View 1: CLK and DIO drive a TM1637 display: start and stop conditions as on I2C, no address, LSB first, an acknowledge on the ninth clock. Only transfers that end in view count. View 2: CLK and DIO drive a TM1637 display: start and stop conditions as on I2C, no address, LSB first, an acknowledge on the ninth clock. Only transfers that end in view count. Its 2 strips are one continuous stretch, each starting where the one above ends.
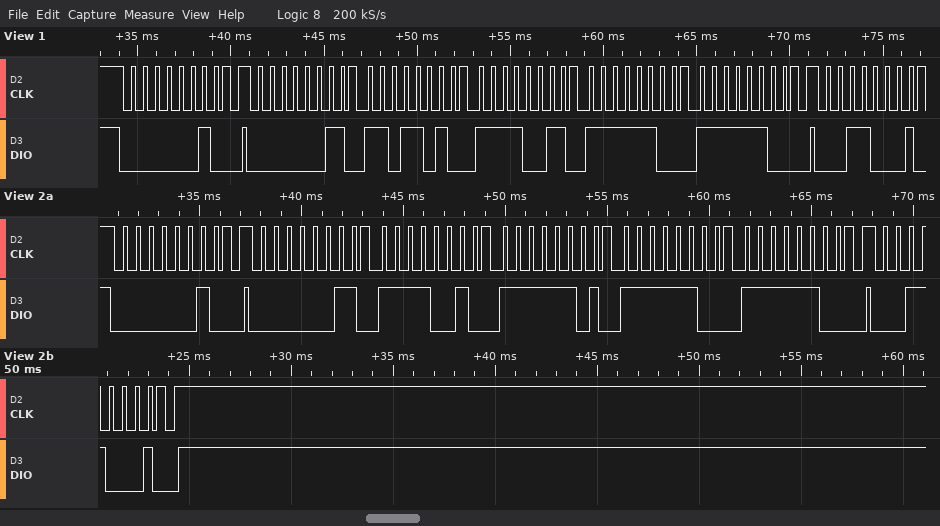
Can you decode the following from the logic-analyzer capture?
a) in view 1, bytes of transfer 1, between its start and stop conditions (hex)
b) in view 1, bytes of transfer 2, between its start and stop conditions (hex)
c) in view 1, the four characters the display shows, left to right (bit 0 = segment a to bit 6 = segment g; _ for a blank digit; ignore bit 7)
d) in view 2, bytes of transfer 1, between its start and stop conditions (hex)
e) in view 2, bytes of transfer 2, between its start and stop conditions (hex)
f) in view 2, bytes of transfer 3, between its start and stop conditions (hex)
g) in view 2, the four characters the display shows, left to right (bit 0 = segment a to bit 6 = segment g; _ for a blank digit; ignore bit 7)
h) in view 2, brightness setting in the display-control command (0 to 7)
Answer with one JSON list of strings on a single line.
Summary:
["40", "C0 5B CF 3F 3F", "2300", "40", "C0 4F BF 3F 3F", "8C", "3000", "4"]
